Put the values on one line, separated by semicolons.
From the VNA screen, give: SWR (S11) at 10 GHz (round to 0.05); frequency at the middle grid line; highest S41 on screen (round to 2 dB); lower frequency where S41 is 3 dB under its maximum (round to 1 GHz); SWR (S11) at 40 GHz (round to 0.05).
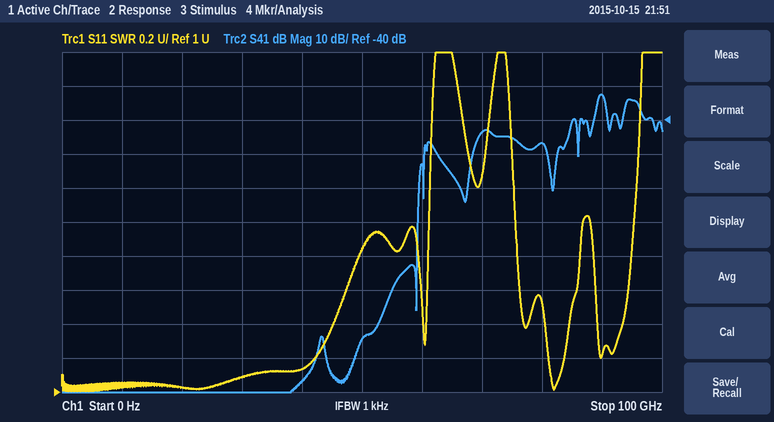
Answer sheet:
1.05; 50 GHz; -32 dB; 89 GHz; 1.15
